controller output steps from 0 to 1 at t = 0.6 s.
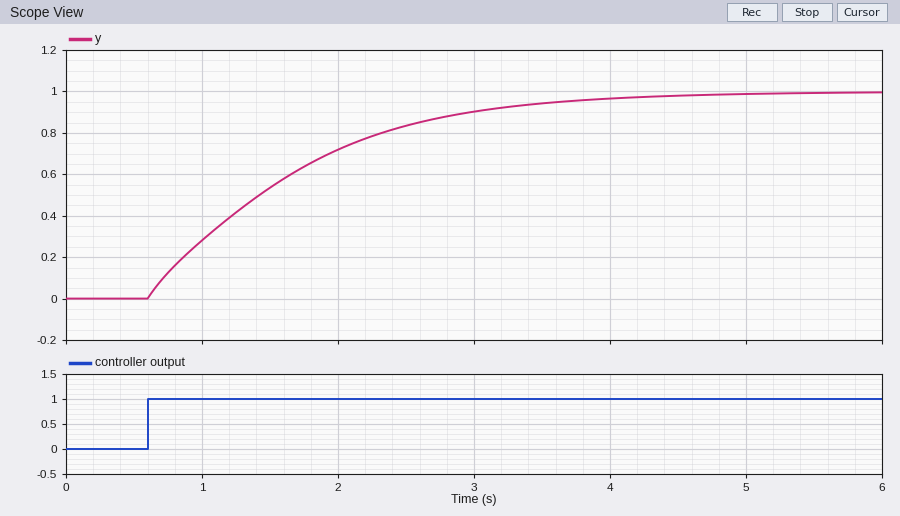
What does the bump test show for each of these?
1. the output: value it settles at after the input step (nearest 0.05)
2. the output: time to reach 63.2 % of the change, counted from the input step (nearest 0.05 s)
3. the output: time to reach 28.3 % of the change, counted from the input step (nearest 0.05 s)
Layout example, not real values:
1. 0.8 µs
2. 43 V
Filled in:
1. 1.00
2. 1.15 s
3. 0.40 s
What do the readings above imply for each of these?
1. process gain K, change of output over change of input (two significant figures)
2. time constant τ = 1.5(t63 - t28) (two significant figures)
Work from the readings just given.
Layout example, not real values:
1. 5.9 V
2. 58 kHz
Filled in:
1. 1.0
2. 1.1 s
